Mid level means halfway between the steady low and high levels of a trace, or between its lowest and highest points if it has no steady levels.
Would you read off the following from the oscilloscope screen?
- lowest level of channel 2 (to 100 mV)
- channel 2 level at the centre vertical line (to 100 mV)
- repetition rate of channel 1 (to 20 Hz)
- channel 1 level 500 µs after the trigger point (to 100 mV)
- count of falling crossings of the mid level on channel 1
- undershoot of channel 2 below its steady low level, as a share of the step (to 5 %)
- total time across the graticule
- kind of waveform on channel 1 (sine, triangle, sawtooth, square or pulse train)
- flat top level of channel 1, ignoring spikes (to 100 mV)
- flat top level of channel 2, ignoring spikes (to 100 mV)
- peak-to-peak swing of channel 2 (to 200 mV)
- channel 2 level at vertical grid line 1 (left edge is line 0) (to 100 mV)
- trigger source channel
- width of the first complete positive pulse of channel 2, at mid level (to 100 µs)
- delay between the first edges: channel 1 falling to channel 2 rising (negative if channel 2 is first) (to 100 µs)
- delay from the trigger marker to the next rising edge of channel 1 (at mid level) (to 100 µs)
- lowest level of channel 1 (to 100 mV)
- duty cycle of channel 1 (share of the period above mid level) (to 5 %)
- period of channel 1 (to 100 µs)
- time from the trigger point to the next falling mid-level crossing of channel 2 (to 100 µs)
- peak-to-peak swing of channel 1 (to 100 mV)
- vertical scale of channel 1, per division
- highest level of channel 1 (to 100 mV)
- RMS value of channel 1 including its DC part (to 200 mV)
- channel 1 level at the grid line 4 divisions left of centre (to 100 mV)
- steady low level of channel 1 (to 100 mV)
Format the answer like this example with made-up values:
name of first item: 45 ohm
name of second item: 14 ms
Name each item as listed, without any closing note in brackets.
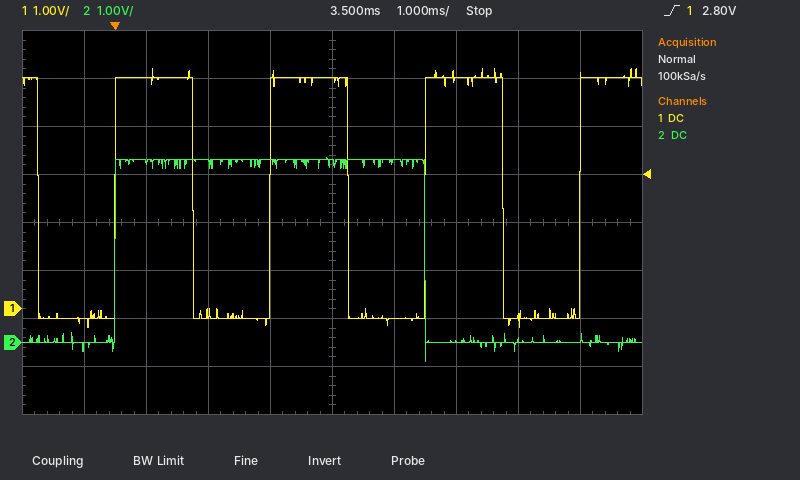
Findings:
lowest level of channel 2: -400 mV
channel 2 level at the centre vertical line: 3.7 V
repetition rate of channel 1: 400 Hz
channel 1 level 500 µs after the trigger point: 4.8 V
count of falling crossings of the mid level on channel 1: 4
undershoot of channel 2 below its steady low level, as a share of the step: 10 %
total time across the graticule: 10 ms
kind of waveform on channel 1: square
flat top level of channel 1, ignoring spikes: 4.8 V
flat top level of channel 2, ignoring spikes: 3.8 V
peak-to-peak swing of channel 2: 4.2 V
channel 2 level at vertical grid line 1 (left edge is line 0): -100 mV
trigger source channel: channel 1
width of the first complete positive pulse of channel 2, at mid level: 5.0 ms
delay between the first edges: channel 1 falling to channel 2 rising (negative if channel 2 is first): +1.2 ms
delay from the trigger marker to the next rising edge of channel 1 (at mid level): 2.5 ms
lowest level of channel 1: -400 mV
duty cycle of channel 1 (share of the period above mid level): 50 %
period of channel 1: 2.5 ms
time from the trigger point to the next falling mid-level crossing of channel 2: 5.0 ms
peak-to-peak swing of channel 1: 5.4 V
vertical scale of channel 1, per division: 1 V
highest level of channel 1: 5.0 V
RMS value of channel 1 including its DC part: 3.4 V
channel 1 level at the grid line 4 divisions left of centre: -200 mV
steady low level of channel 1: -200 mV
